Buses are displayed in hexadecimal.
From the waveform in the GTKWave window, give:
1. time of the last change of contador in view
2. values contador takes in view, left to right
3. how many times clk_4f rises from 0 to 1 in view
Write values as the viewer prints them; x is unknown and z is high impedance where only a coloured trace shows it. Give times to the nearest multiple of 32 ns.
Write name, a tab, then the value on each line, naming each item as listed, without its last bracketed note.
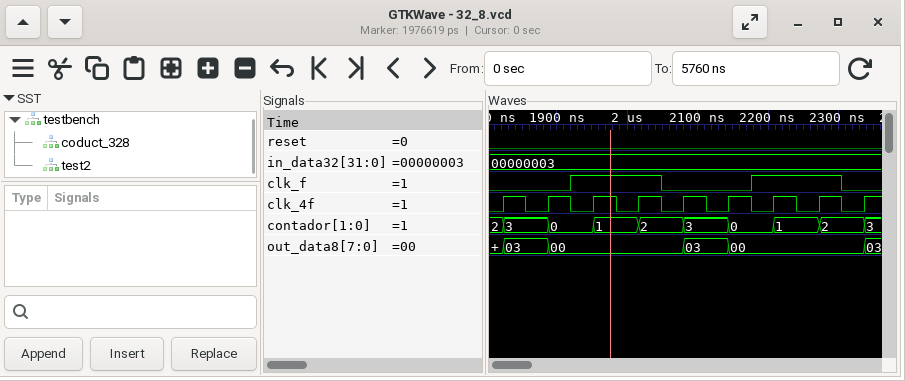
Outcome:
time of the last change of contador in view	2336 ns
values contador takes in view, left to right	2, 3, 0, 1, 2, 3, 0, 1, 2, 3
how many times clk_4f rises from 0 to 1 in view	9
